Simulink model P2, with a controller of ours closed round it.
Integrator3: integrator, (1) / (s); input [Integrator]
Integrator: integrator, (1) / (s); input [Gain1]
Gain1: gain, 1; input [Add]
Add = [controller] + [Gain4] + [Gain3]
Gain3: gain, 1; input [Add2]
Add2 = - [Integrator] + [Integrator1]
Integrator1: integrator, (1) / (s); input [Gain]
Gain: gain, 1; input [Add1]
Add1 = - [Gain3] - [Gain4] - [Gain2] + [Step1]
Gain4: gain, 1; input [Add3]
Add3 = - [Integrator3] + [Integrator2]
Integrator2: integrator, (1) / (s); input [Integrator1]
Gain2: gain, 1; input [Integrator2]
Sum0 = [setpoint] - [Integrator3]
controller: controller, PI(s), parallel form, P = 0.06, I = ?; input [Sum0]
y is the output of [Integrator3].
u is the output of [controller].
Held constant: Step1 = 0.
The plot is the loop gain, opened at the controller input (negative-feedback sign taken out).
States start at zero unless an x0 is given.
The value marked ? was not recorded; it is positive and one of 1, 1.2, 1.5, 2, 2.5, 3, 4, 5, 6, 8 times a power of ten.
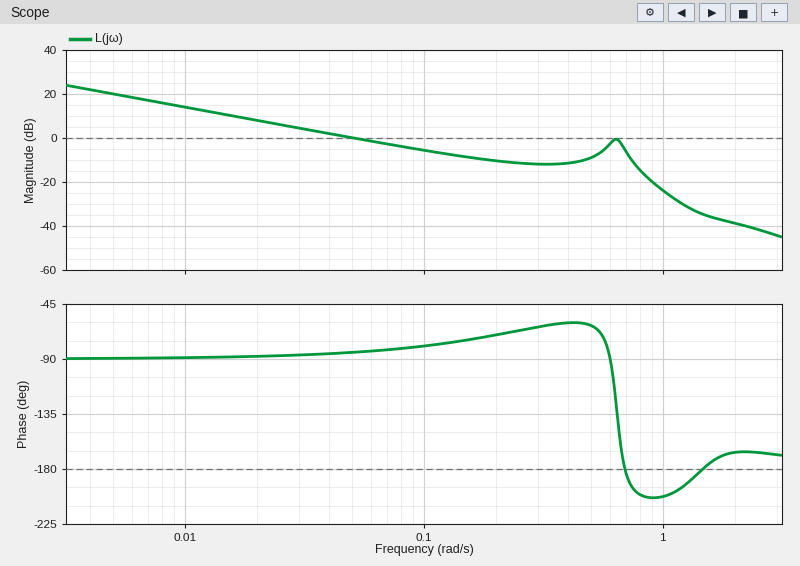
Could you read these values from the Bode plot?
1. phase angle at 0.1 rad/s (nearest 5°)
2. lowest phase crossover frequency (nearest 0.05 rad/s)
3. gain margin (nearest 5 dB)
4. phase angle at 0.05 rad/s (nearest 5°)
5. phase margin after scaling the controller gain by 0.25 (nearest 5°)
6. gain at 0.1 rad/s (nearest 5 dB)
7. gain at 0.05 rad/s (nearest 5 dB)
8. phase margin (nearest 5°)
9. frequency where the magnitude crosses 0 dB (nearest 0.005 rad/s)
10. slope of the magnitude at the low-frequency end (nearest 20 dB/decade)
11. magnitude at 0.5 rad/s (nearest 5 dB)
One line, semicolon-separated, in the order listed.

-80°; 0.70 rad/s; 5 dB; -85°; 90°; -5 dB; 0 dB; 95°; 0.050 rad/s; -20 dB/decade; -10 dB
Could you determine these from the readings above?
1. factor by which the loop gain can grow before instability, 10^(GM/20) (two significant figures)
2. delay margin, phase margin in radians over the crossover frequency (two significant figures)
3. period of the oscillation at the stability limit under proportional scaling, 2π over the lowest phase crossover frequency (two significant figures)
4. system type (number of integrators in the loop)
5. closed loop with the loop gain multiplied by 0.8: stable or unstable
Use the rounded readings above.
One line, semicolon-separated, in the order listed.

1.8; 33 s; 9.0 s; 1; stable
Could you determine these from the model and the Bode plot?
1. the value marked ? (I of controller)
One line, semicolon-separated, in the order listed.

0.025
